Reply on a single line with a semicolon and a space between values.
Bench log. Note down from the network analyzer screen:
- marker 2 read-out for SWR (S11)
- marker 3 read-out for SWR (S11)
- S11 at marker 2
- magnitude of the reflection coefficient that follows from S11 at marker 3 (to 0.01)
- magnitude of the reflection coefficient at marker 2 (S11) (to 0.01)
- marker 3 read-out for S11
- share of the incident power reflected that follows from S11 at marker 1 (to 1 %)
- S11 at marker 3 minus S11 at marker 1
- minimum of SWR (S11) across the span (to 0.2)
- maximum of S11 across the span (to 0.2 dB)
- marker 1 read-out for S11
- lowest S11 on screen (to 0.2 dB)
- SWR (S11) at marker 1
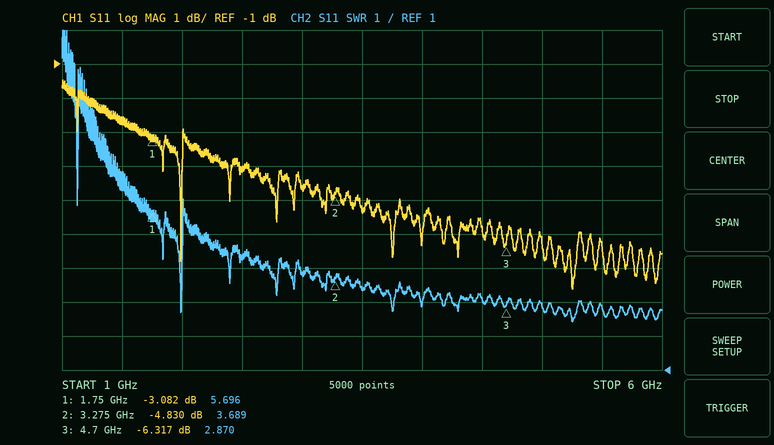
3.689; 2.870; -4.830 dB; 0.48; 0.57; -6.317 dB; 49 %; -3.235 dB; 2.4; -1.4 dB; -3.082 dB; -7.6 dB; 5.696
